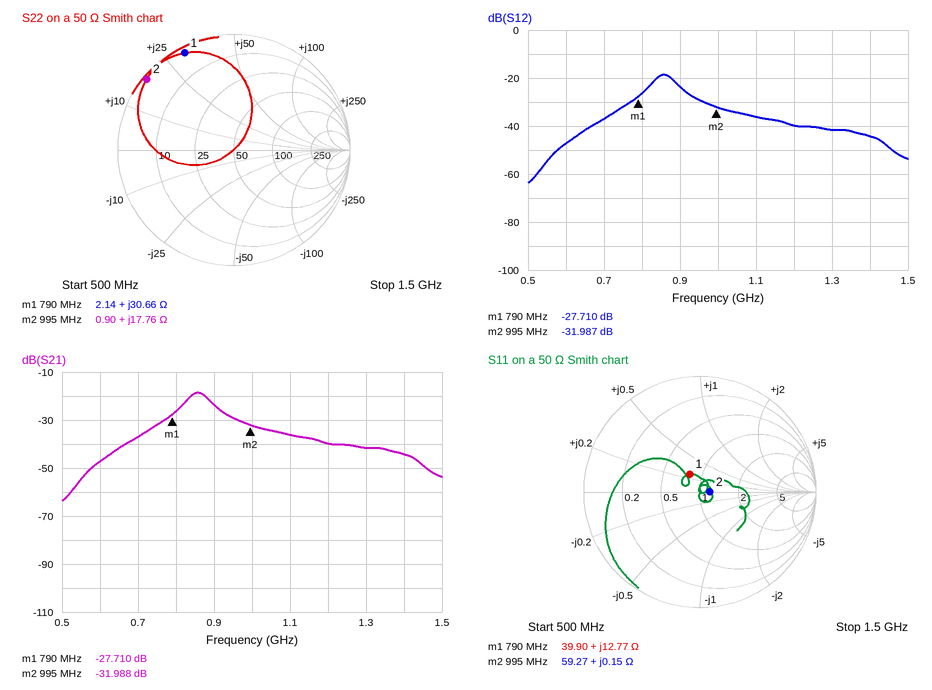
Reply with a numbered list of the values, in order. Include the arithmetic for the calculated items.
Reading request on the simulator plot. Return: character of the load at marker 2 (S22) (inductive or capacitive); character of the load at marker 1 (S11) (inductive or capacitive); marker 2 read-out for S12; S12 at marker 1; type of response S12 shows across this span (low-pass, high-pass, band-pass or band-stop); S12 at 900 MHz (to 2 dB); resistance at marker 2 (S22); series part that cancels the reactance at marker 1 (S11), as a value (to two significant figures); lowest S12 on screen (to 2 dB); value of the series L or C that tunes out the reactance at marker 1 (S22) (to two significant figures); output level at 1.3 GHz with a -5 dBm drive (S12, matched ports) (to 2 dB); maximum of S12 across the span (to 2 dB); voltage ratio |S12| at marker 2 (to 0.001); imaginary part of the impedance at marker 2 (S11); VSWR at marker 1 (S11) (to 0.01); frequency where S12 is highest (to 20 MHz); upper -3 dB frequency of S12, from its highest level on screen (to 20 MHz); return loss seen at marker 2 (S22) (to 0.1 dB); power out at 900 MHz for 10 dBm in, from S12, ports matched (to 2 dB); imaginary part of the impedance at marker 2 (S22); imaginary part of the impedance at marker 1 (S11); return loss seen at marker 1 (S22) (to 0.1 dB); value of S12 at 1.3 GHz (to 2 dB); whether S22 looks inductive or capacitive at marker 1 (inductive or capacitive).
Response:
1. inductive
2. inductive
3. -31.987 dB
4. -27.710 dB
5. band-pass
6. -24 dB
7. 0.90 Ω
8. C = 1/(2π × 790 MHz × 12.77 Ω) ≈ 16 pF
9. -64 dB
10. C = 1/(2π × 790 MHz × 30.66 Ω) ≈ 6.6 pF
11. -5 dBm + (-42 dB) = -46 dBm
12. -18 dB
13. 10^(-31.987/20) ≈ 0.025
14. +0.15 Ω
15. 1.44
16. 860 MHz
17. 880 MHz
18. 0.3 dB
19. 10 dBm + (-24 dB) = -14 dBm
20. +17.76 Ω
21. +12.77 Ω
22. 0.5 dB
23. -42 dB
24. inductive
